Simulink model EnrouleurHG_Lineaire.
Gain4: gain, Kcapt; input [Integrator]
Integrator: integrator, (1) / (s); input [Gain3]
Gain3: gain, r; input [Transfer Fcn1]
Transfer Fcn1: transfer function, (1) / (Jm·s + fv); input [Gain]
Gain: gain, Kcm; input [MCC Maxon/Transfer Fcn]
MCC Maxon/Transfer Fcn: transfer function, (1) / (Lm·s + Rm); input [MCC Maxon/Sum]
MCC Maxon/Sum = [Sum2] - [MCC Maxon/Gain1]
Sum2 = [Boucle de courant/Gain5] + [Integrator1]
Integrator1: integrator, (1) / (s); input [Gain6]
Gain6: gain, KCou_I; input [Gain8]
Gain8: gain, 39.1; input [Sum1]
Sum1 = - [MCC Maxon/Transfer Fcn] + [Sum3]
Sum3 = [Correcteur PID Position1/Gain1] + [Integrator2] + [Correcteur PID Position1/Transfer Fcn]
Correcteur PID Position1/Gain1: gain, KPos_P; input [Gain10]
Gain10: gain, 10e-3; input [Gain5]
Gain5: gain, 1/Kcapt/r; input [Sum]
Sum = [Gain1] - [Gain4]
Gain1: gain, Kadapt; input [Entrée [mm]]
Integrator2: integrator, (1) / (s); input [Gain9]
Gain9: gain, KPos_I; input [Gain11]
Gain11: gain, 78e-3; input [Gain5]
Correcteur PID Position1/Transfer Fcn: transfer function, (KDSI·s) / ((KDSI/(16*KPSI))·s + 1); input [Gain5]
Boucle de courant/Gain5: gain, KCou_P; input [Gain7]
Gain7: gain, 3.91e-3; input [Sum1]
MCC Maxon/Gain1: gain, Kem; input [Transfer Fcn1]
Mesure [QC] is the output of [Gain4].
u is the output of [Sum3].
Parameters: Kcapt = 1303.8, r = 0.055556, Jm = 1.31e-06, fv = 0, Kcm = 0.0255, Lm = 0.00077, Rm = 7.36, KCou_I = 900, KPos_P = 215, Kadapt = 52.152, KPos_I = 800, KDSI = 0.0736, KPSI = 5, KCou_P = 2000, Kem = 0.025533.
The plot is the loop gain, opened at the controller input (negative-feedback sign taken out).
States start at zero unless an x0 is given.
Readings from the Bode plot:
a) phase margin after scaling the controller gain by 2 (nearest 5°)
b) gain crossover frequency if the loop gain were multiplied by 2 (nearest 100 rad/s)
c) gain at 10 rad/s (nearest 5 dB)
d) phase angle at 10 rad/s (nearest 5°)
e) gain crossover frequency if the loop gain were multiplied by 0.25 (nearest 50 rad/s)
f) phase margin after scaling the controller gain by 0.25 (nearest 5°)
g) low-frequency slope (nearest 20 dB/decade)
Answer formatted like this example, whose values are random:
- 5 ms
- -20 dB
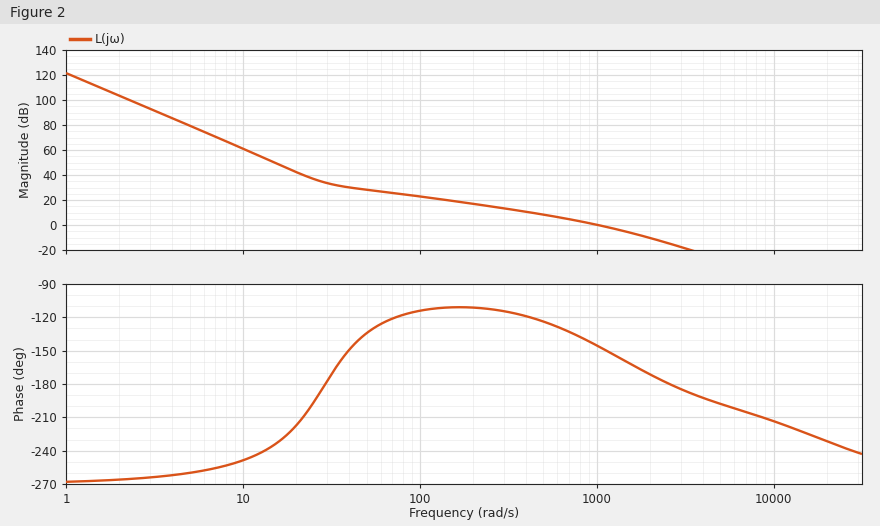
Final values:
- 20°
- 1500 rad/s
- 60 dB
- -250°
- 350 rad/s
- 65°
- -60 dB/decade
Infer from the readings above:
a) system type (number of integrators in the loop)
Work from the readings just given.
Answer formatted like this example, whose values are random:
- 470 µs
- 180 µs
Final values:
- 3
